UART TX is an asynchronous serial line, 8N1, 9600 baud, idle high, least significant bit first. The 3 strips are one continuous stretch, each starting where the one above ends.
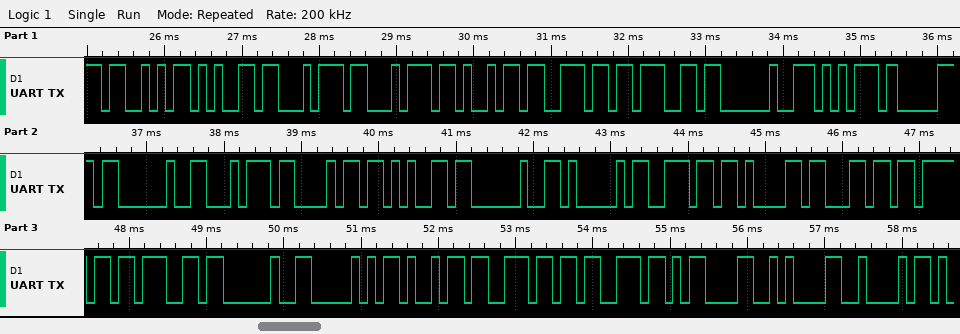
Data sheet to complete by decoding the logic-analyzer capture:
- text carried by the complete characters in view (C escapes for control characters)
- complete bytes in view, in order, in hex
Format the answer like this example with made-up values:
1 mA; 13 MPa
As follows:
"Setting up the Analog Pins\r\nB"; 53 65 74 74 69 6E 67 20 75 70 20 74 68 65 20 41 6E 61 6C 6F 67 20 50 69 6E 73 0D 0A 42
